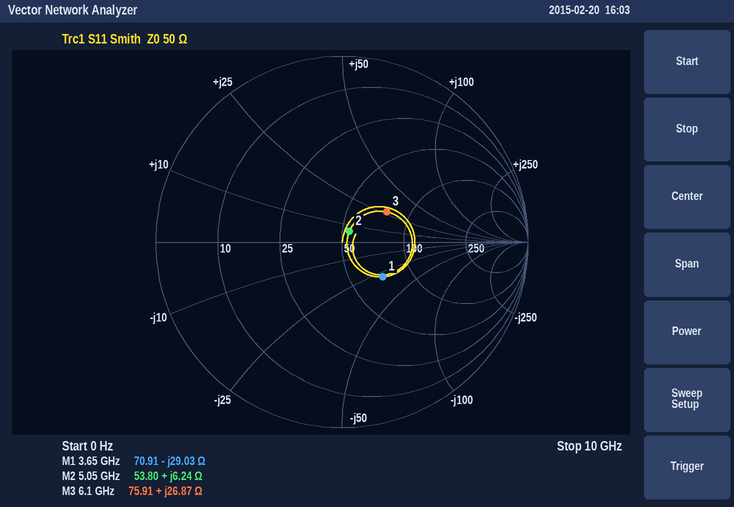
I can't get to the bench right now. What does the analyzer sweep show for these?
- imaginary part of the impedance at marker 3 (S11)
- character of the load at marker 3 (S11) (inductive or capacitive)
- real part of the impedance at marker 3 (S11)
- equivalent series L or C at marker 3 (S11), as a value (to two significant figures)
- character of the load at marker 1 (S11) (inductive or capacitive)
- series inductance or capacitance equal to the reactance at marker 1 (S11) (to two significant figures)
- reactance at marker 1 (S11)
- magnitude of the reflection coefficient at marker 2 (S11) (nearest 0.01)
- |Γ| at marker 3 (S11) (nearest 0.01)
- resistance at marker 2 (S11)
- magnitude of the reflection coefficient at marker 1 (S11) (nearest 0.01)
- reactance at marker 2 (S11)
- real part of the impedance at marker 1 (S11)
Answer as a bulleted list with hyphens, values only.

- +26.87 Ω
- inductive
- 75.91 Ω
- 700 pH
- capacitive
- 1.5 pF
- -29.03 Ω
- 0.07
- 0.29
- 53.80 Ω
- 0.29
- +6.24 Ω
- 70.91 Ω
